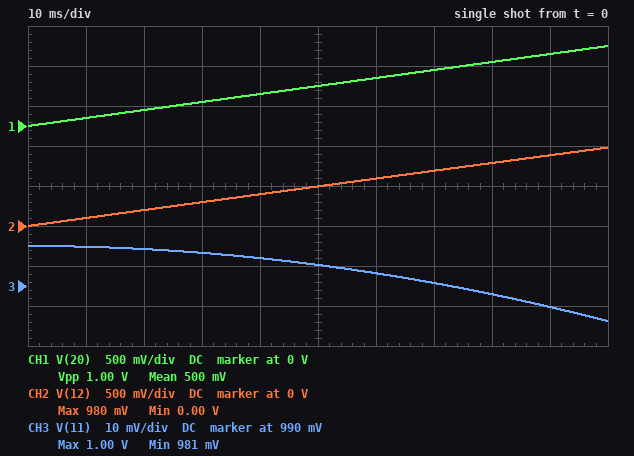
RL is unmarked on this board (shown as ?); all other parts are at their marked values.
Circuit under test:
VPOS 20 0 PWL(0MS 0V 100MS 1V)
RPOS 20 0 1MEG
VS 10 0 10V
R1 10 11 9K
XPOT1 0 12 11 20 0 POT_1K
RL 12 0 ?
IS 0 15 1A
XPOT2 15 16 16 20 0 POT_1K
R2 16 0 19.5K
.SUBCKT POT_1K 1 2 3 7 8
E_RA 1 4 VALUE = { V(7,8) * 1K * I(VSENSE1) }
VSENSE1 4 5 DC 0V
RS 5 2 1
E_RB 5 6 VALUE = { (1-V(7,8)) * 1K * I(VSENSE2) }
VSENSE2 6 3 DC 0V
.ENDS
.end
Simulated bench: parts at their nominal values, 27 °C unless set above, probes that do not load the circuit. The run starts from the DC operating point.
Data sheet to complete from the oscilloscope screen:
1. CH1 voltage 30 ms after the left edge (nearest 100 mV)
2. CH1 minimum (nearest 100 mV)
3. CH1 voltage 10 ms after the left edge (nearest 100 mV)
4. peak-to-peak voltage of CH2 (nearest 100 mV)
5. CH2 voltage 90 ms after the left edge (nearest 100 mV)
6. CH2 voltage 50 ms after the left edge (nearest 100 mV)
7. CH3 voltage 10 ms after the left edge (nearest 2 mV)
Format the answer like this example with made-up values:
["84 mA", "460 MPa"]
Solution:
["300 mV", "0 V", "100 mV", "1.0 V", "900 mV", "500 mV", "1.000 V"]
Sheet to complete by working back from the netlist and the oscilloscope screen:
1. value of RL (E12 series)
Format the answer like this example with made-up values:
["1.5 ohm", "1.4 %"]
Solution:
["47 kΩ"]
